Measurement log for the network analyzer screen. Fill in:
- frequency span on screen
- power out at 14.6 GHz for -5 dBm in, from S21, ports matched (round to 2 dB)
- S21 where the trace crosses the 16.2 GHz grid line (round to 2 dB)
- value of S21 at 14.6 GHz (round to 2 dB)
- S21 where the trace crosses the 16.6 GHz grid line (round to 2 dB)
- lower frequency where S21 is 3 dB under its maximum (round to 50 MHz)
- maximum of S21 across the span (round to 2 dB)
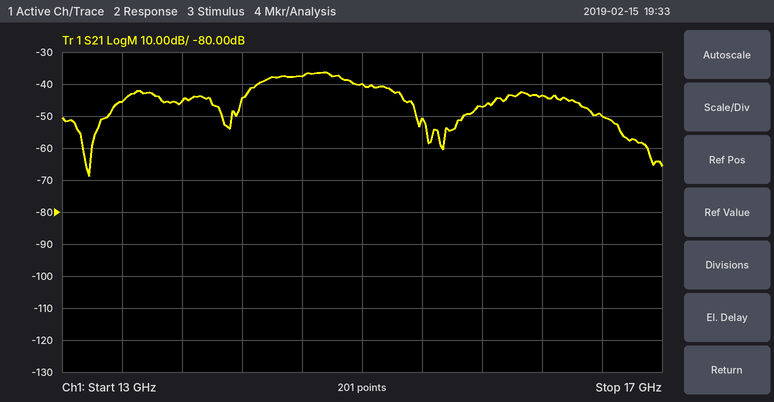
4 GHz
-42 dBm
-44 dB
-38 dB
-50 dB
14.30 GHz
-36 dB
